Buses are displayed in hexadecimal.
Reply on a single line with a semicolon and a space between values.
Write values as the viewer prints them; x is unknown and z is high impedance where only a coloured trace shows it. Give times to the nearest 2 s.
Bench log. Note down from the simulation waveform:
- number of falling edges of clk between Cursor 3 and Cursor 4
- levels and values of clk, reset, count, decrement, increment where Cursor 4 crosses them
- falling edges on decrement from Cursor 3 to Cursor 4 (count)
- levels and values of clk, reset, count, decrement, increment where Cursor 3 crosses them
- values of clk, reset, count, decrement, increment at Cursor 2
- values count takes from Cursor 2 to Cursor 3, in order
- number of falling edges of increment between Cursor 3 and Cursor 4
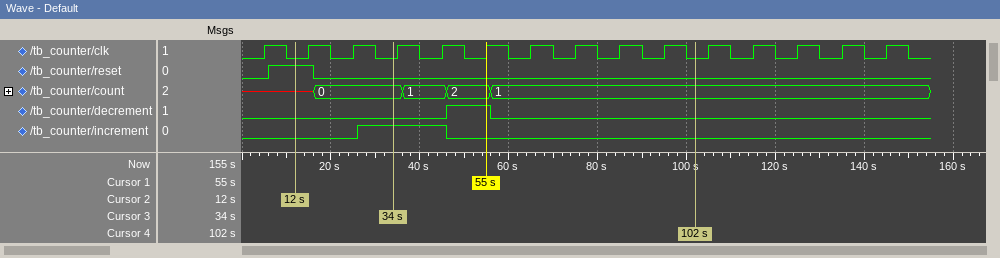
7; clk=0, reset=0, count=1, decrement=0, increment=0; 1; clk=0, reset=0, count=0, decrement=0, increment=1; clk=0, reset=1, count=x, decrement=0, increment=0; x, 0; 1
